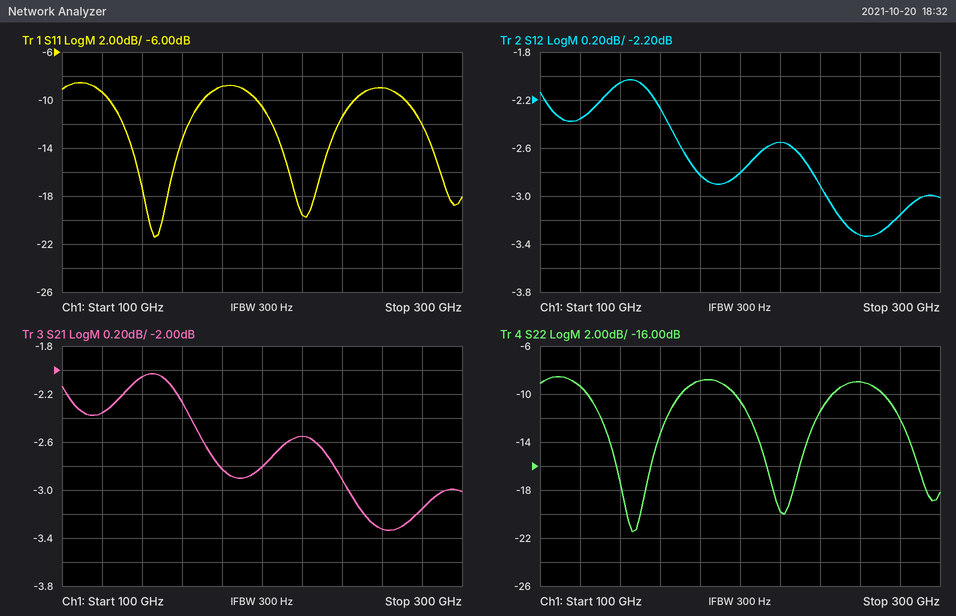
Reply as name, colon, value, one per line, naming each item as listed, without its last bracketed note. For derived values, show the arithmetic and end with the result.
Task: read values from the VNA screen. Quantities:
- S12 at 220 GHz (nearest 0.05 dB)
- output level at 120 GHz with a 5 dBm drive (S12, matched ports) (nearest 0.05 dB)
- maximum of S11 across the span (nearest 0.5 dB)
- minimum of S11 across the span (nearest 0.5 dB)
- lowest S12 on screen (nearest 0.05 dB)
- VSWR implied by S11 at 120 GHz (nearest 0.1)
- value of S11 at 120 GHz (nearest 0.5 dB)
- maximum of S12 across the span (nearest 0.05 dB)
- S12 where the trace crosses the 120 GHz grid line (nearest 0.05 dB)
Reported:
S12 at 220 GHz: -2.55 dB
output level at 120 GHz with a 5 dBm drive (S12, matched ports): 5 dBm + (-2.35 dB) = 2.65 dBm
maximum of S11 across the span: -8.5 dB
minimum of S11 across the span: -21.5 dB
lowest S12 on screen: -3.35 dB
VSWR implied by S11 at 120 GHz: |Γ| = 10^(-9.5/20) = 0.3350; VSWR = (1 + 0.3350)/(1 − 0.3350) ≈ 2.0
value of S11 at 120 GHz: -9.5 dB
maximum of S12 across the span: -2.05 dB
S12 where the trace crosses the 120 GHz grid line: -2.35 dB
